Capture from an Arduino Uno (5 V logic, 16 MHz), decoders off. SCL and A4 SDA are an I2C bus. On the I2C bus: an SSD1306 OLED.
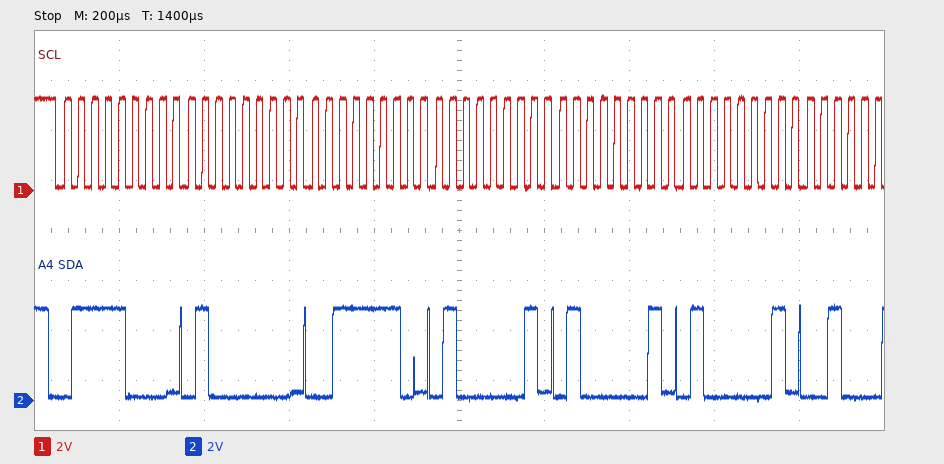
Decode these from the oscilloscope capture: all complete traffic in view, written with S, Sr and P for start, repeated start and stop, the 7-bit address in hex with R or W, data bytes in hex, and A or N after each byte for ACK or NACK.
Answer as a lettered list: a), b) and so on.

a) S 3CW A 40 A 3E A 41 A 41 A 41 A
